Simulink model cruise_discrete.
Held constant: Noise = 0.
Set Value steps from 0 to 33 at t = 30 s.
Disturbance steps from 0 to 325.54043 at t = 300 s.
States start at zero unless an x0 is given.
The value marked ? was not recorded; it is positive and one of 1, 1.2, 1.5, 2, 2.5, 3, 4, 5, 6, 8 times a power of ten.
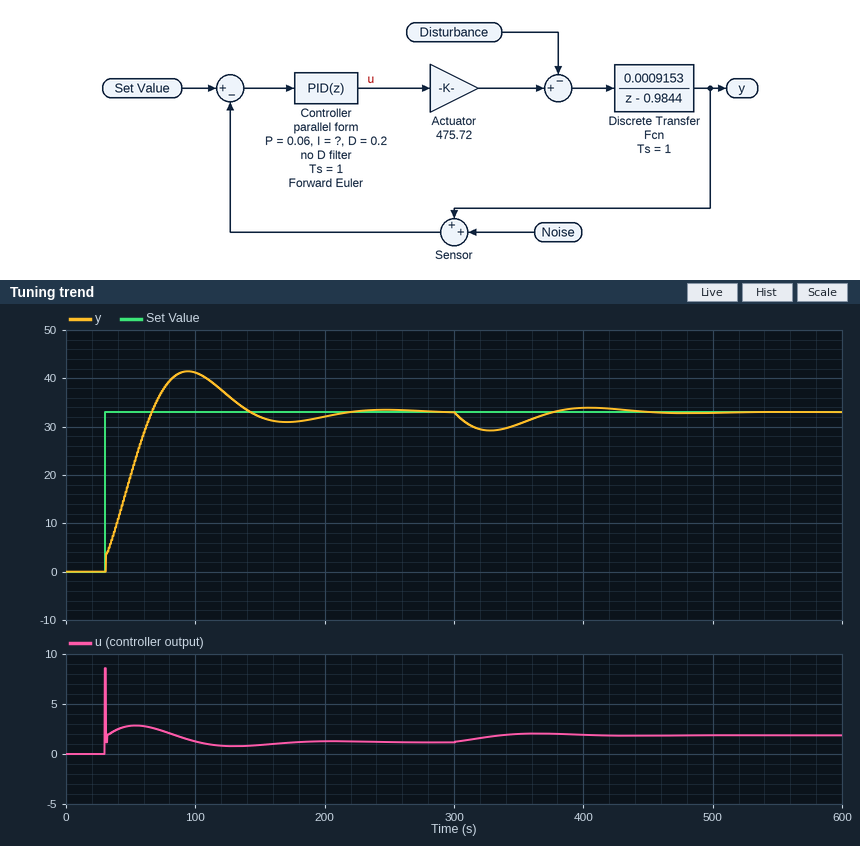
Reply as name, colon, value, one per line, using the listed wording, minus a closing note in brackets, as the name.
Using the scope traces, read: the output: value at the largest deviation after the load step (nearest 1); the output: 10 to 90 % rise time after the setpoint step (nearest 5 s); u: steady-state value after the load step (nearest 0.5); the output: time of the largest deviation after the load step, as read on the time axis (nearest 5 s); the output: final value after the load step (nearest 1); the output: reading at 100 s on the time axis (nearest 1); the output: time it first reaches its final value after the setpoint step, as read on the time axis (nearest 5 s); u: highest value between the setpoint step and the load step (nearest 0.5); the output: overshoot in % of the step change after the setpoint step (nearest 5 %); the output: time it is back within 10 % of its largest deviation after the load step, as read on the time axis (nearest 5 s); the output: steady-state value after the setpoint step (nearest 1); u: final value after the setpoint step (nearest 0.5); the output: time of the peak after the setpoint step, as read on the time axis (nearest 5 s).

the output: value at the largest deviation after the load step: 29
the output: 10 to 90 % rise time after the setpoint step: 30 s
u: steady-state value after the load step: 2.0
the output: time of the largest deviation after the load step, as read on the time axis: 330 s
the output: final value after the load step: 33
the output: reading at 100 s on the time axis: 41
the output: time it first reaches its final value after the setpoint step, as read on the time axis: 65 s
u: highest value between the setpoint step and the load step: 8.5
the output: overshoot in % of the step change after the setpoint step: 25 %
the output: time it is back within 10 % of its largest deviation after the load step, as read on the time axis: 435 s
the output: steady-state value after the setpoint step: 33
u: final value after the setpoint step: 1.0
the output: time of the peak after the setpoint step, as read on the time axis: 95 s
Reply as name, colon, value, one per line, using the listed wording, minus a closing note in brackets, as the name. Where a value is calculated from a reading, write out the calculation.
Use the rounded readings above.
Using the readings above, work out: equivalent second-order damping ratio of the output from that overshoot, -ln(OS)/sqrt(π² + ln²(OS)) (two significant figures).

equivalent second-order damping ratio of the output from that overshoot, -ln(OS)/sqrt(π² + ln²(OS)): ln(0.25) = -1.386; 1.386 / sqrt(9.870 + 1.922) = 0.40
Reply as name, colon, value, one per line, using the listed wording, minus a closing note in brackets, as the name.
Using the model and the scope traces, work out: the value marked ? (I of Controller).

the value marked ?: 0.005
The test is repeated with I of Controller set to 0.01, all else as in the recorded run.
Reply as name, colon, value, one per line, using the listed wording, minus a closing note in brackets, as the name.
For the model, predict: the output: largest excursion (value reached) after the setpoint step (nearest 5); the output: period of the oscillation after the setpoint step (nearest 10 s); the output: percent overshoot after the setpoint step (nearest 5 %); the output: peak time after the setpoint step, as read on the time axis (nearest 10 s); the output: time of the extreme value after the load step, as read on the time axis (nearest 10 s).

the output: largest excursion (value reached) after the setpoint step: 45
the output: period of the oscillation after the setpoint step: 100 s
the output: percent overshoot after the setpoint step: 40 %
the output: peak time after the setpoint step, as read on the time axis: 80 s
the output: time of the extreme value after the load step, as read on the time axis: 320 s
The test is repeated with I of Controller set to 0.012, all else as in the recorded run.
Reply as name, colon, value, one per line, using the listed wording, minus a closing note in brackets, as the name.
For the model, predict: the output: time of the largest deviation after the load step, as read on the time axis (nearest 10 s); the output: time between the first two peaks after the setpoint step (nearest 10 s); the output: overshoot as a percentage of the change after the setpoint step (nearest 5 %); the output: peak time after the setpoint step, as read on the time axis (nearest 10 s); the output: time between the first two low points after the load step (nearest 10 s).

the output: time of the largest deviation after the load step, as read on the time axis: 320 s
the output: time between the first two peaks after the setpoint step: 90 s
the output: overshoot as a percentage of the change after the setpoint step: 45 %
the output: peak time after the setpoint step, as read on the time axis: 70 s
the output: time between the first two low points after the load step: 90 s
